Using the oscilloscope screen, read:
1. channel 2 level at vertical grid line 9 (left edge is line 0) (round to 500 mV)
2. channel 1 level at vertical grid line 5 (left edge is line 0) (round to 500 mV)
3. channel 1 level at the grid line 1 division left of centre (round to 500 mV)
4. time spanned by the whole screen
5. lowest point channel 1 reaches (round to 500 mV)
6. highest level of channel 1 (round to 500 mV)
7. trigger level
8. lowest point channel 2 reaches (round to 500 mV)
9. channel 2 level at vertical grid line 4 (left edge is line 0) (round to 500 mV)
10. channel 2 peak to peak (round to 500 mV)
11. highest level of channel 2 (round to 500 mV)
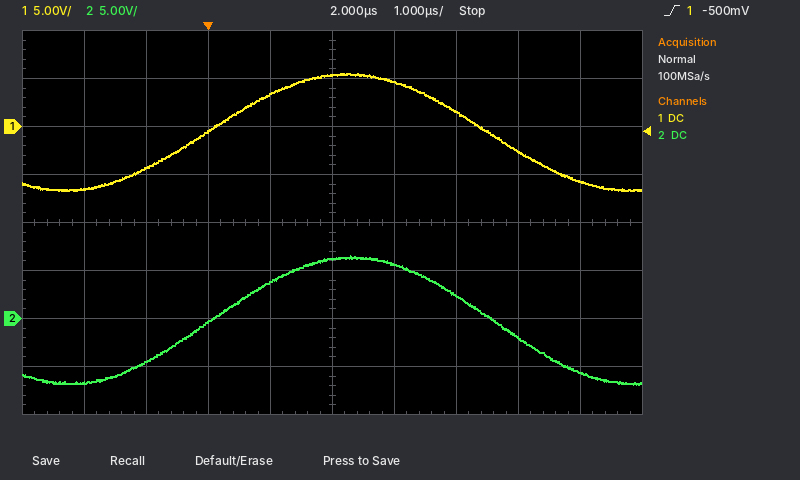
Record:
-5.5 V
5.5 V
3.5 V
10 µs
-6.5 V
5.5 V
-500 mV
-7.0 V
4.0 V
13.5 V
6.5 V
